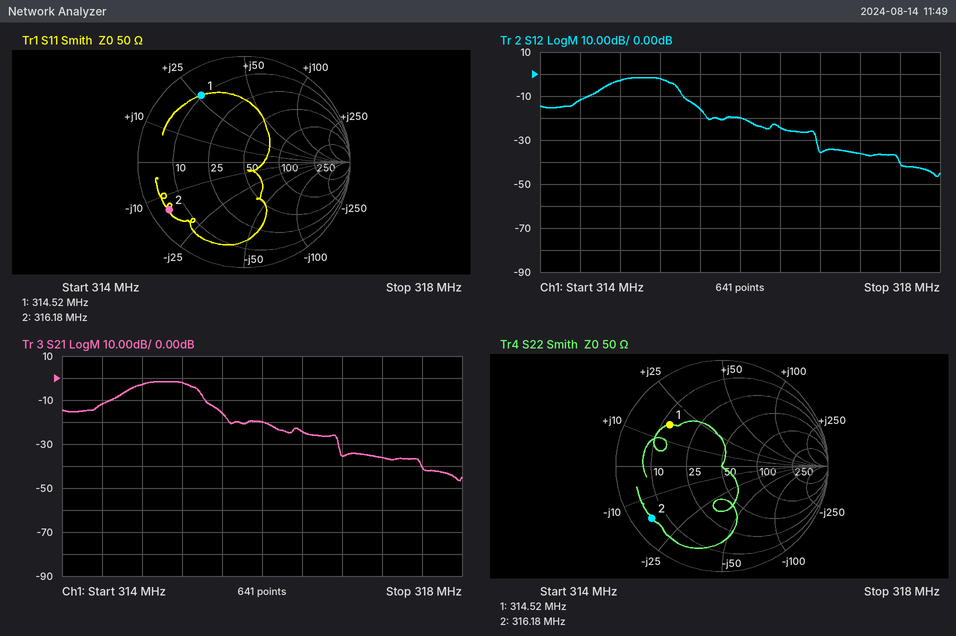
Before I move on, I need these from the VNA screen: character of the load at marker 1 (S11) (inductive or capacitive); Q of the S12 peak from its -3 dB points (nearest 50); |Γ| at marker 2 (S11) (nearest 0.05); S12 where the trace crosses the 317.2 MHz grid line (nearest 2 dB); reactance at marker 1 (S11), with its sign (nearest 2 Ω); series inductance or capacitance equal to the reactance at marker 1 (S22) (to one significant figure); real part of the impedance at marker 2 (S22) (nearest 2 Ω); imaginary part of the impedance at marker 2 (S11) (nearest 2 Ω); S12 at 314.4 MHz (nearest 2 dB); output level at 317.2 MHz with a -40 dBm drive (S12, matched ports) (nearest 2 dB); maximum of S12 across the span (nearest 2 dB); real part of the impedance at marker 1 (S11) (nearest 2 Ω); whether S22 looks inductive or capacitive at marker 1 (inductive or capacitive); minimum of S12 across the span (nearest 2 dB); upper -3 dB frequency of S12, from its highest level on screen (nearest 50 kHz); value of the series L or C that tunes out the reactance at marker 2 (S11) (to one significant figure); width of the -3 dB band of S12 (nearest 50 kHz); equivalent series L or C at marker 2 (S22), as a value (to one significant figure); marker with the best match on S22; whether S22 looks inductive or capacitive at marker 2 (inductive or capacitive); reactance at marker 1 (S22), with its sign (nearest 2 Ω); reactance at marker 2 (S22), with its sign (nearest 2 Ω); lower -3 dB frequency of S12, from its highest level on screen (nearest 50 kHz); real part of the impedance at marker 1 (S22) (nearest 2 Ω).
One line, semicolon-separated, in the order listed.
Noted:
inductive; 500; 0.85; -36 dB; +26 Ω; 8 nH; 6 Ω; -14 Ω; -12 dB; -76 dBm; -2 dB; 10 Ω; inductive; -46 dB; 315.35 MHz; 7 nH; 650 kHz; 30 pF; marker 1; capacitive; +16 Ω; -16 Ω; 314.70 MHz; 12 Ω
